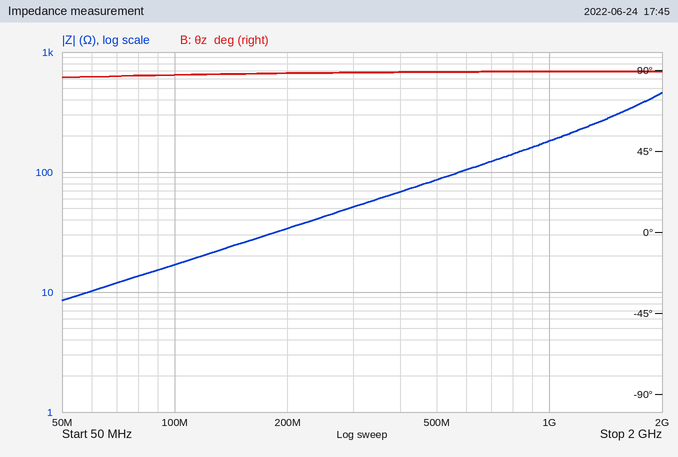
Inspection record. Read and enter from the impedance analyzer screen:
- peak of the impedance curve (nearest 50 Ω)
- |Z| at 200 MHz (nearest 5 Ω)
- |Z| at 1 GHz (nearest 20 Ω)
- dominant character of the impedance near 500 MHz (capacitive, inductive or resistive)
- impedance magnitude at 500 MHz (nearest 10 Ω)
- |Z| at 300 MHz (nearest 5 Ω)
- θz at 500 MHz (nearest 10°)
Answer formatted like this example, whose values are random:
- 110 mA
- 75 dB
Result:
- 450 Ω
- 35 Ω
- 180 Ω
- inductive
- 90 Ω
- 50 Ω
- 90°
